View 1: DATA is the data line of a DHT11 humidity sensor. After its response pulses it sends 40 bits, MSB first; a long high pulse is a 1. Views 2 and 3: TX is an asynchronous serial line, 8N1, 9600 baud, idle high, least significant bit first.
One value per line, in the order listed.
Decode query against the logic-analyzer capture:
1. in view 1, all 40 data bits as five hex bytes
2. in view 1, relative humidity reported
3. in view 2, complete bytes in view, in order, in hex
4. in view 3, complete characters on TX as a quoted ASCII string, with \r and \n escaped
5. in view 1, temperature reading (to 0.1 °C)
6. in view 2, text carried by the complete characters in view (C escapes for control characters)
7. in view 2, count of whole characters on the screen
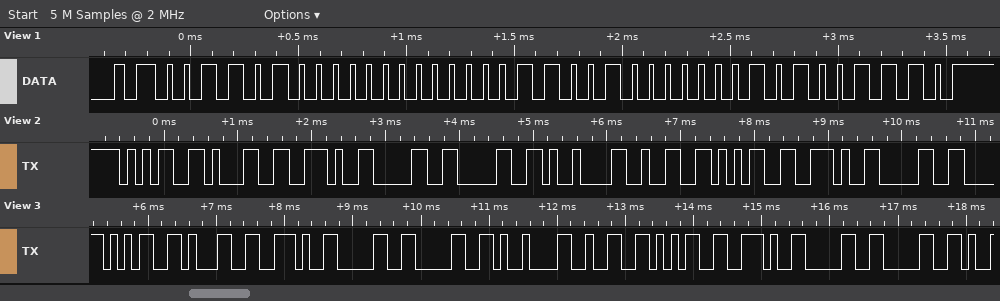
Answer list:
34 00 19 01 4E
52 %
35 31 2E 30 30 09 32 35 2E 30
"51.00\t25.00"
25.1 °C
"51.00\t25.0"
10
